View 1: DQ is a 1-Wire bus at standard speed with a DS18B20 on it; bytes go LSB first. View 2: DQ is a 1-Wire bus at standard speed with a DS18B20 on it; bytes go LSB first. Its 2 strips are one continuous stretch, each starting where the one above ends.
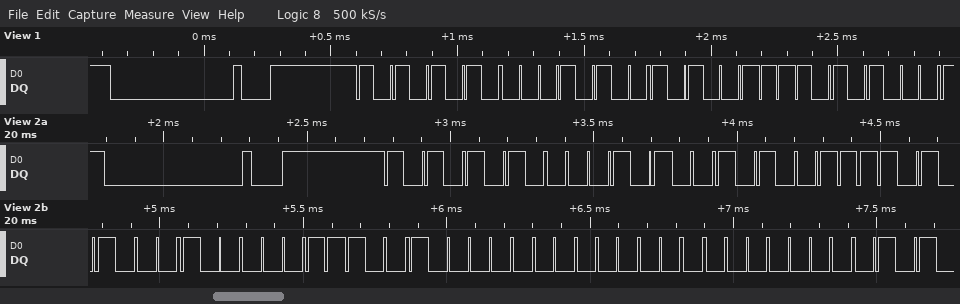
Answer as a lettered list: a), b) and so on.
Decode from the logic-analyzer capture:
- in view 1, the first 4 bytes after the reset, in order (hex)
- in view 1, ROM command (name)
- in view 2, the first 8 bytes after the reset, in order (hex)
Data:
a) 55 28 E5 15
b) Match ROM
c) 55 28 E5 15 C1 09 00 00
